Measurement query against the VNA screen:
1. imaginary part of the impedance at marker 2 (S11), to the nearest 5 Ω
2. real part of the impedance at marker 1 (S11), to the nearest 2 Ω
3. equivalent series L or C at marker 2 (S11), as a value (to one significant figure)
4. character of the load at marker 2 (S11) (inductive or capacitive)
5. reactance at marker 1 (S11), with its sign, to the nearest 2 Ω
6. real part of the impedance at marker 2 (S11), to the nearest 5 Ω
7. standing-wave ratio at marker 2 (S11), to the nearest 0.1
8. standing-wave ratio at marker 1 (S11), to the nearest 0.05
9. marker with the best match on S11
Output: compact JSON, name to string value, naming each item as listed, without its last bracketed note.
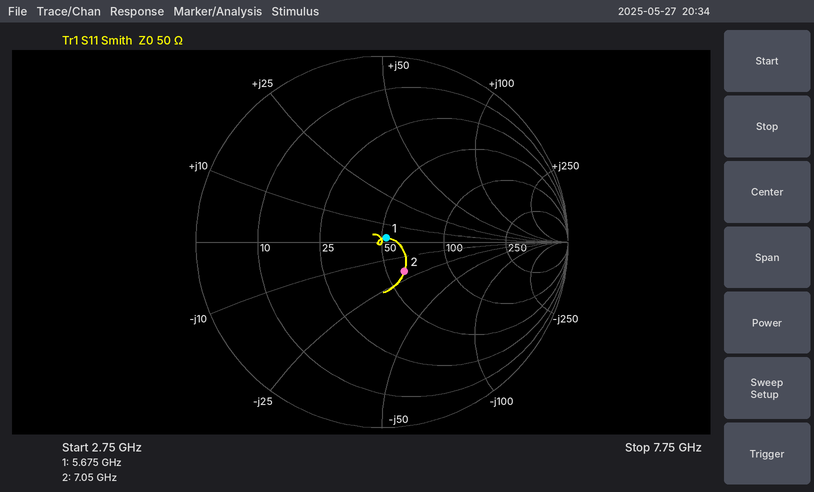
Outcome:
{"imaginary part of the impedance at marker 2 (S11), to the nearest 5 Ω": "-20 Ω", "real part of the impedance at marker 1 (S11), to the nearest 2 Ω": "52 Ω", "equivalent series L or C at marker 2 (S11), as a value": "1 pF", "character of the load at marker 2 (S11)": "capacitive", "reactance at marker 1 (S11), with its sign, to the nearest 2 Ω": "+2 Ω", "real part of the impedance at marker 2 (S11), to the nearest 5 Ω": "60 Ω", "standing-wave ratio at marker 2 (S11), to the nearest 0.1": "1.5", "standing-wave ratio at marker 1 (S11), to the nearest 0.05": "1.05", "marker with the best match on S11": "marker 1"}
